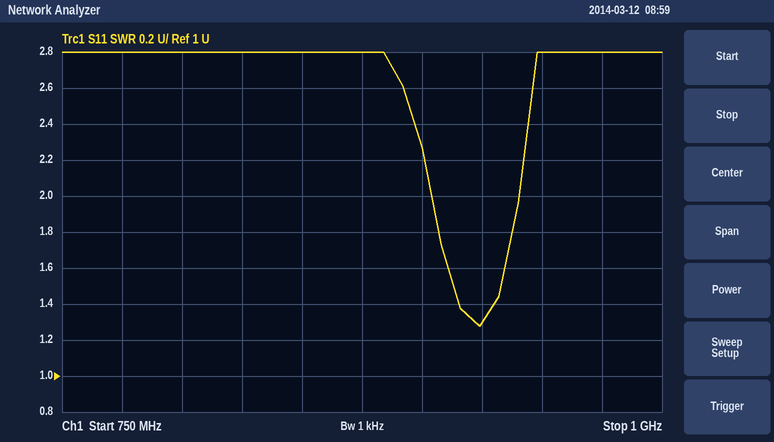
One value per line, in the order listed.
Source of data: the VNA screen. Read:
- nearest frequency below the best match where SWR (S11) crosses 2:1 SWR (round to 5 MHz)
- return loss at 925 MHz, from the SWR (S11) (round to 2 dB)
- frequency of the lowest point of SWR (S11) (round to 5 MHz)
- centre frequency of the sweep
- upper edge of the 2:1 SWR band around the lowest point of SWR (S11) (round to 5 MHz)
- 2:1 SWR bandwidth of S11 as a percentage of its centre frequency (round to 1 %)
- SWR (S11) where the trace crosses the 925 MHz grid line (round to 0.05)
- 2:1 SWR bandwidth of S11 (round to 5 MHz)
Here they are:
905 MHz
18 dB
925 MHz
875 MHz
940 MHz
4 %
1.30
35 MHz
